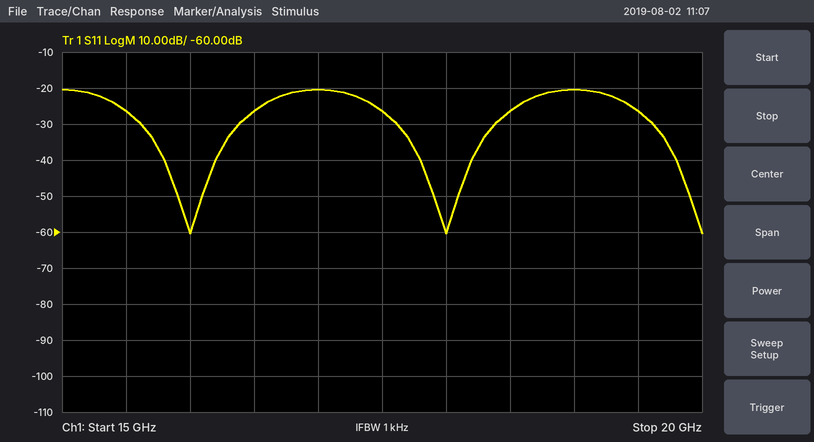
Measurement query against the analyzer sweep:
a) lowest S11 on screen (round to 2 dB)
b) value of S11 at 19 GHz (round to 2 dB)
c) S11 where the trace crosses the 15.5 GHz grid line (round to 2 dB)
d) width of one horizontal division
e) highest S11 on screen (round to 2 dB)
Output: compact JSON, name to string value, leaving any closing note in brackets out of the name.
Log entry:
{"lowest S11 on screen": "-60 dB", "value of S11 at 19 GHz": "-20 dB", "S11 where the trace crosses the 15.5 GHz grid line": "-26 dB", "width of one horizontal division": "500 MHz", "highest S11 on screen": "-20 dB"}
